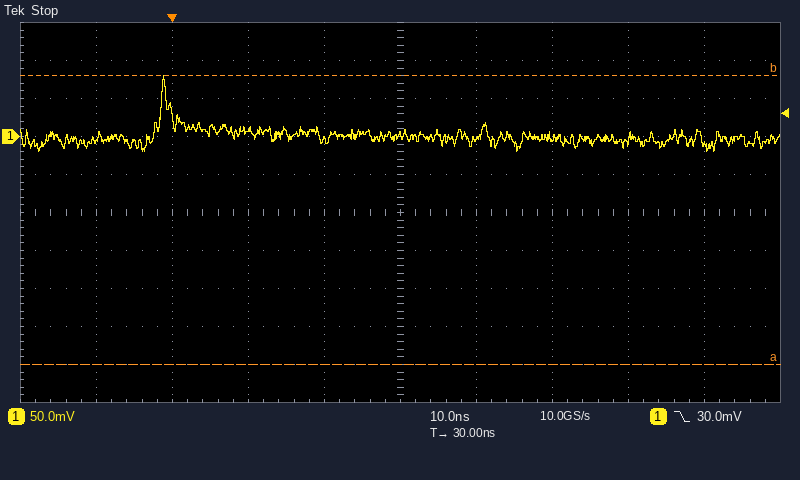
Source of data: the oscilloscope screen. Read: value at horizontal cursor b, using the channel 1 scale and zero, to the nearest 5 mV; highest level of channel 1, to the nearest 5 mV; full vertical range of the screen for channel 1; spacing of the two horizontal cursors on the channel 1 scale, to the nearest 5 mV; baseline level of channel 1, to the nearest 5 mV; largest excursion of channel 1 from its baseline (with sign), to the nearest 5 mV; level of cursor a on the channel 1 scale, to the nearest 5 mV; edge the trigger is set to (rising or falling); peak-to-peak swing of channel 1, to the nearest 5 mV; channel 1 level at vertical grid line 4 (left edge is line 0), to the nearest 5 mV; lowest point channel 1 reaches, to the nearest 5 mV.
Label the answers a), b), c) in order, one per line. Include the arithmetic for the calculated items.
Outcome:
a) 80 mV
b) 80 mV
c) 500 mV
d) 380 mV
e) 0 mV
f) 80 mV − (0 mV) = +80 mV
g) -300 mV
h) falling
i) 80 mV − (-20 mV) = 100 mV
j) -5 mV
k) -20 mV
